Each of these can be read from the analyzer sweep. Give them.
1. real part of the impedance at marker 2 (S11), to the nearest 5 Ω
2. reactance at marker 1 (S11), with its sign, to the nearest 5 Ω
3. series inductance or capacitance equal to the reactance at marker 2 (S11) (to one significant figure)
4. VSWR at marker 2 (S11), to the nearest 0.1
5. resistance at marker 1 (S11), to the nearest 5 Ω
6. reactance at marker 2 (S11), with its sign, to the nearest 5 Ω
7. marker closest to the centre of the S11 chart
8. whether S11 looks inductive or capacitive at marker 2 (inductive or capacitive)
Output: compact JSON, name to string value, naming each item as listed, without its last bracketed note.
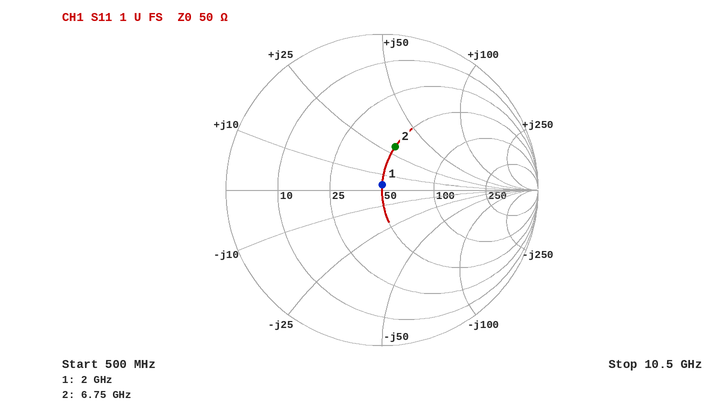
{"real part of the impedance at marker 2 (S11), to the nearest 5 Ω": "50 Ω", "reactance at marker 1 (S11), with its sign, to the nearest 5 Ω": "+5 Ω", "series inductance or capacitance equal to the reactance at marker 2 (S11)": "700 pH", "VSWR at marker 2 (S11), to the nearest 0.1": "1.8", "resistance at marker 1 (S11), to the nearest 5 Ω": "50 Ω", "reactance at marker 2 (S11), with its sign, to the nearest 5 Ω": "+30 Ω", "marker closest to the centre of the S11 chart": "marker 1", "whether S11 looks inductive or capacitive at marker 2": "inductive"}
